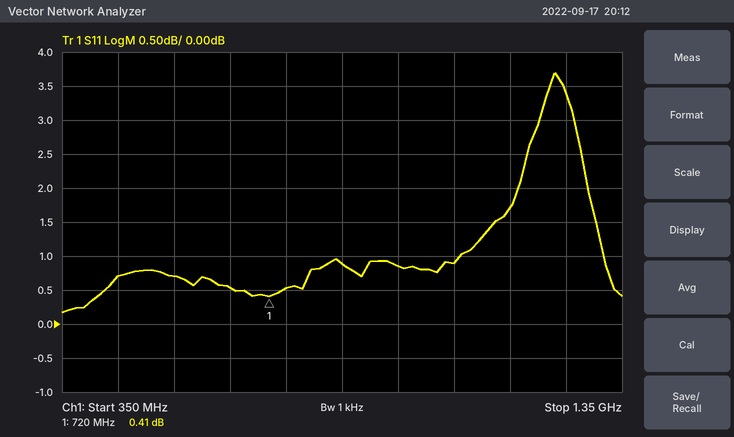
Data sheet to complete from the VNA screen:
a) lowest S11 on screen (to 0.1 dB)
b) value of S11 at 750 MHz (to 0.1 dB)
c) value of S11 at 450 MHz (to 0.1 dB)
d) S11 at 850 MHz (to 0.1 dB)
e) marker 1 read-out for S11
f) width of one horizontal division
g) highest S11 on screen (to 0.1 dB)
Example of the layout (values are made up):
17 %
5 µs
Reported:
0.2 dB
0.5 dB
0.7 dB
0.9 dB
0.41 dB
100 MHz
3.7 dB
